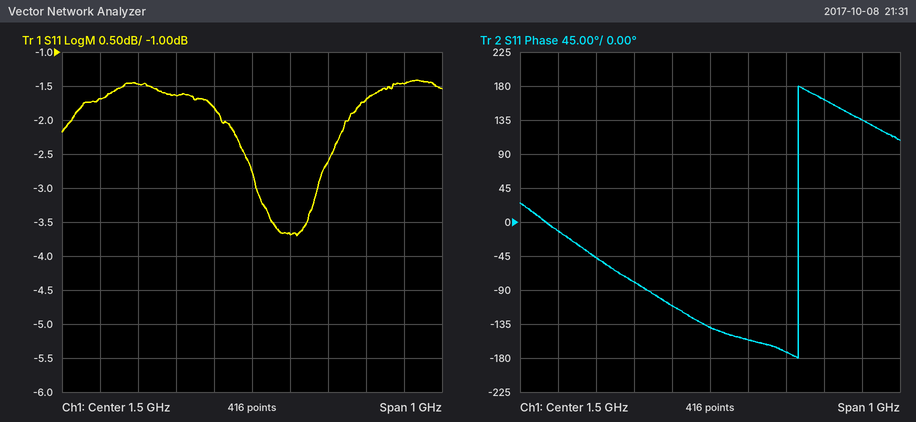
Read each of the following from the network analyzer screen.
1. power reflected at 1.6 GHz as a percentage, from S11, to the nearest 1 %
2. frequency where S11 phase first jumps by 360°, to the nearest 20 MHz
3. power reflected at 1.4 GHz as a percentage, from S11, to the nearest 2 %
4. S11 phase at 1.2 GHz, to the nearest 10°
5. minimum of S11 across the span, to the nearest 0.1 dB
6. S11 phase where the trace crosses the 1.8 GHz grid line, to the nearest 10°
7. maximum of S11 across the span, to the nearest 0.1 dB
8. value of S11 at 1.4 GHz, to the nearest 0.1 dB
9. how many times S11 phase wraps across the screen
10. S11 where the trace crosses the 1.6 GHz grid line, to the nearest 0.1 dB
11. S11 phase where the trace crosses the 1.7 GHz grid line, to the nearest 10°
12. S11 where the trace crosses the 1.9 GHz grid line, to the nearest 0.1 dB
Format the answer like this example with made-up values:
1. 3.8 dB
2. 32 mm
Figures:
1. 43 %
2. 1.74 GHz
3. 66 %
4. -50°
5. -3.7 dB
6. 160°
7. -1.4 dB
8. -1.8 dB
9. 1
10. -3.7 dB
11. -170°
12. -1.5 dB
